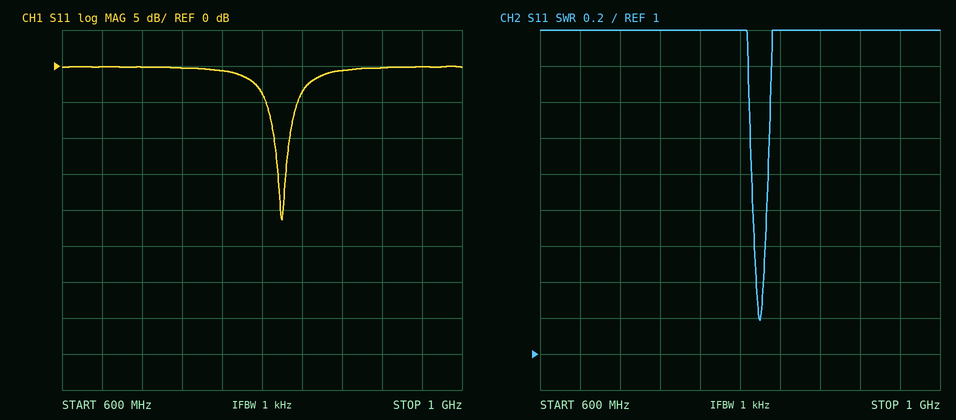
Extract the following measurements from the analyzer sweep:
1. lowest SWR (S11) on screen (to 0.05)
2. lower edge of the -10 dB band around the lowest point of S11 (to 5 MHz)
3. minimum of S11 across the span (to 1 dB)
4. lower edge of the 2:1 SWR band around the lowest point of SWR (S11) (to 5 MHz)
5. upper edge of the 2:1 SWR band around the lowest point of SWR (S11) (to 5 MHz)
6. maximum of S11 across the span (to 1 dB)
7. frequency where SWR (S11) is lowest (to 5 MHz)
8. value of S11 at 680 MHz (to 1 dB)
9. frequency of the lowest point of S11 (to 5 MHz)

1.20
810 MHz
-21 dB
810 MHz
830 MHz
0 dB
820 MHz
0 dB
820 MHz
